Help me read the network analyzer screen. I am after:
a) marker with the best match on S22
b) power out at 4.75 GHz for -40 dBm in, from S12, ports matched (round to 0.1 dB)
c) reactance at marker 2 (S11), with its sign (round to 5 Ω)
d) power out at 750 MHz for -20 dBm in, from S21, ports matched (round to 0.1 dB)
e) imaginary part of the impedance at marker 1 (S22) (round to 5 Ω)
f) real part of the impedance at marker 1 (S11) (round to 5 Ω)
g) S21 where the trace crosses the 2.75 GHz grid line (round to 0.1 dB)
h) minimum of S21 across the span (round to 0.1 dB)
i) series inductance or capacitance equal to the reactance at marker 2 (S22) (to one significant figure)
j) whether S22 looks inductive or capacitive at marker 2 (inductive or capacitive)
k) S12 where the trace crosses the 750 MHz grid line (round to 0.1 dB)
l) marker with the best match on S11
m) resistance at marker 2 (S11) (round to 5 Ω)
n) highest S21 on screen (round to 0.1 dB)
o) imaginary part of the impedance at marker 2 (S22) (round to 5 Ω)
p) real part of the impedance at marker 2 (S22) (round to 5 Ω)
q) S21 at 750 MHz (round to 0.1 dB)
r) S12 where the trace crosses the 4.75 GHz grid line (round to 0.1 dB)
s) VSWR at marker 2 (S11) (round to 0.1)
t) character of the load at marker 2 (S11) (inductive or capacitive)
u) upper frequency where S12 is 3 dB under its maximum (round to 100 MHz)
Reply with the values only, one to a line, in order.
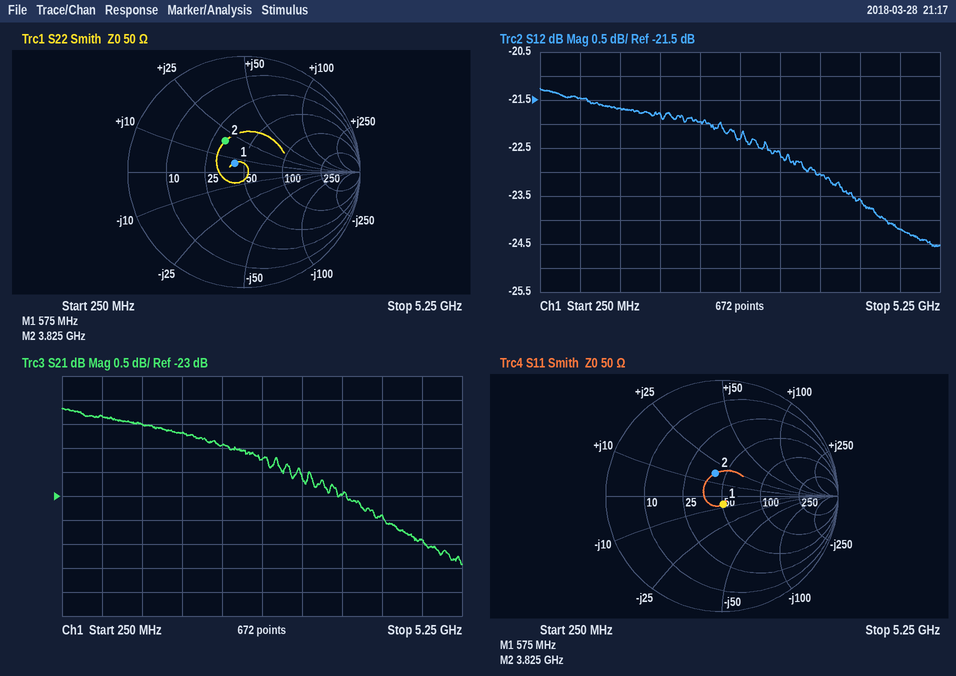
marker 1
-64.2 dBm
+15 Ω
-41.3 dBm
+5 Ω
50 Ω
-22.2 dB
-24.4 dB
800 pH
inductive
-21.5 dB
marker 1
40 Ω
-21.2 dB
+20 Ω
30 Ω
-21.3 dB
-24.2 dB
1.5
inductive
4.8 GHz
